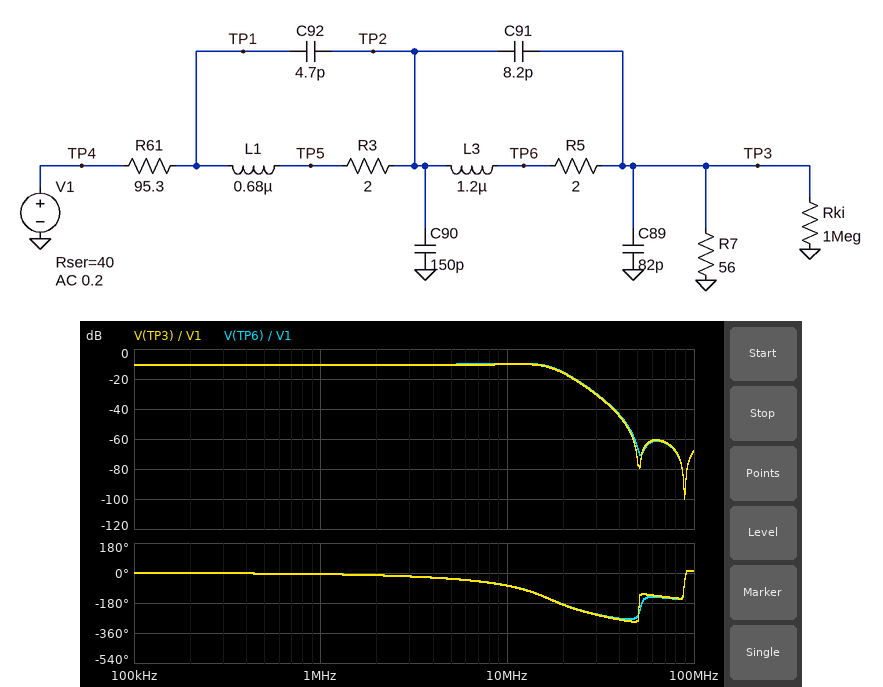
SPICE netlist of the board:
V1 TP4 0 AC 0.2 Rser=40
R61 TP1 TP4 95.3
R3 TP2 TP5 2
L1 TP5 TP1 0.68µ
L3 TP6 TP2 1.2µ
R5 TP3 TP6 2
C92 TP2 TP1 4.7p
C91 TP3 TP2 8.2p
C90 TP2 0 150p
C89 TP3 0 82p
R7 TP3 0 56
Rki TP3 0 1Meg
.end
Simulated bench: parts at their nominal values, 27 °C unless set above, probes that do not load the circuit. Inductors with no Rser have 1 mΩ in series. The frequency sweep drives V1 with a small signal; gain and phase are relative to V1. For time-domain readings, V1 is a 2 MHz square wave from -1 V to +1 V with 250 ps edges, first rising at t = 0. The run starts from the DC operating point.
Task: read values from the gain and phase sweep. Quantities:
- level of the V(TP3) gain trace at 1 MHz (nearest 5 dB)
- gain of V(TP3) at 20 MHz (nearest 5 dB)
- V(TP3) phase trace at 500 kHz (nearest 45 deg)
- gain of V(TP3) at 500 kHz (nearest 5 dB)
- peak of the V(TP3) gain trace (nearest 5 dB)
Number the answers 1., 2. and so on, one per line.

1. -10 dB
2. -15 dB
3. 0 deg
4. -10 dB
5. -10 dB
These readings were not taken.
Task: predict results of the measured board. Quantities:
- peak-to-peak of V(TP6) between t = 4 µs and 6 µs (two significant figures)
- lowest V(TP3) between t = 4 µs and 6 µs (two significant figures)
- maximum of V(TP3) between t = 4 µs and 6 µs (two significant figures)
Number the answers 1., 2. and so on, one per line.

1. 790 mV
2. -380 mV
3. 380 mV
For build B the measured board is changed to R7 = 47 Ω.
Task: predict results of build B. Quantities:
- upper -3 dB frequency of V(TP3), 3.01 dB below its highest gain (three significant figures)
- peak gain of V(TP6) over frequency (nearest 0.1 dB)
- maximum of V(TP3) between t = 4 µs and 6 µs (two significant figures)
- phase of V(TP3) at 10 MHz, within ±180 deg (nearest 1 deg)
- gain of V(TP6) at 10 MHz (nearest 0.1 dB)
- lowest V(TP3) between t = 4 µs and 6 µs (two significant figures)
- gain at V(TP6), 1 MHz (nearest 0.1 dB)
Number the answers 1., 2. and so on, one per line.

1. 17.3 MHz
2. -10.6 dB
3. 340 mV
4. -75 deg
5. -10.7 dB
6. -340 mV
7. -11.6 dB
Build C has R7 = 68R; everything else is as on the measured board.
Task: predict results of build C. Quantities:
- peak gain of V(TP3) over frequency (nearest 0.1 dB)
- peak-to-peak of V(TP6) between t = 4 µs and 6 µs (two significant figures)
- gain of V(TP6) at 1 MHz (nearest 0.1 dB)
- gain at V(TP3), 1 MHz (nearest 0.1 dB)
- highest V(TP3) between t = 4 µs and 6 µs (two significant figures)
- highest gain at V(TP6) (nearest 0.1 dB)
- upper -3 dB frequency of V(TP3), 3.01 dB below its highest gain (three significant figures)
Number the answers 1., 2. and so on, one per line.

1. -9.3 dB
2. 880 mV
3. -9.4 dB
4. -9.7 dB
5. 430 mV
6. -9.0 dB
7. 18.2 MHz
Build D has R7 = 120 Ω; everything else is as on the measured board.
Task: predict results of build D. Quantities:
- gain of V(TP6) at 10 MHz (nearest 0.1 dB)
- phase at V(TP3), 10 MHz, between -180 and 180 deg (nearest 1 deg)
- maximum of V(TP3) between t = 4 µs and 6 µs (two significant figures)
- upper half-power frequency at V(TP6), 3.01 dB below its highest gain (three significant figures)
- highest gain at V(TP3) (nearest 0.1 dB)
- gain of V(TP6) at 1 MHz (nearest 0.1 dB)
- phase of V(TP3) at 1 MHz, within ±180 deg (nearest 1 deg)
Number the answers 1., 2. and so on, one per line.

1. -7.1 dB
2. -79 deg
3. 560 mV
4. 19.5 MHz
5. -6.7 dB
6. -6.6 dB
7. -8 deg
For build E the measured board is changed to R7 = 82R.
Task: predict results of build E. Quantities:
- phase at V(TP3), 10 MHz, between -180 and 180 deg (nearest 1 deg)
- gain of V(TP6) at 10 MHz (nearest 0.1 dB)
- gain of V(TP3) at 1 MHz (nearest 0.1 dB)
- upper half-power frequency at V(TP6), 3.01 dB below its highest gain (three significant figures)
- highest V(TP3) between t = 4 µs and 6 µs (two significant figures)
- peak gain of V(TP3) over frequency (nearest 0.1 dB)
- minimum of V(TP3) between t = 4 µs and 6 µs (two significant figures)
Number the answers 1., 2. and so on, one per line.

1. -78 deg
2. -8.3 dB
3. -8.6 dB
4. 18.7 MHz
5. 470 mV
6. -8.5 dB
7. -470 mV
